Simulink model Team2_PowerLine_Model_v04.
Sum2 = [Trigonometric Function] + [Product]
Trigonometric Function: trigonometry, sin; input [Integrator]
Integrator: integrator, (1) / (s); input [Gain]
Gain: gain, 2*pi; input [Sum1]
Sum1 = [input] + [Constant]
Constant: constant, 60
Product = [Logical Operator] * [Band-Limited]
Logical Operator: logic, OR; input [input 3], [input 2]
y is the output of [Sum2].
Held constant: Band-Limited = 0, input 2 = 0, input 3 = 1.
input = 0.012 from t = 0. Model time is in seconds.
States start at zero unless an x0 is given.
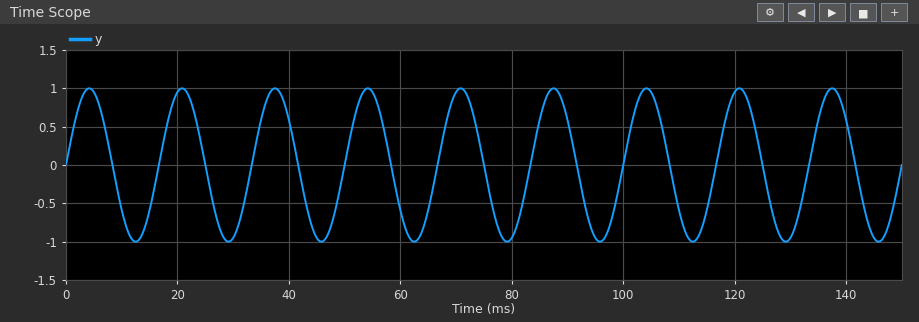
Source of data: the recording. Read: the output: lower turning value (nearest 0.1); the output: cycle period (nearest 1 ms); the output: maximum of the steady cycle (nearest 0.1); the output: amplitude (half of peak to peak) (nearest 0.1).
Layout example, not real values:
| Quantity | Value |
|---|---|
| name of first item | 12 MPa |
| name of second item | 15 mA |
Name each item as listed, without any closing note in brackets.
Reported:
| Quantity | Value |
|---|---|
| the output: lower turning value | -1.0 |
| the output: cycle period | 17 ms |
| the output: maximum of the steady cycle | 1.0 |
| the output: amplitude (half of peak to peak) | 1.0 |
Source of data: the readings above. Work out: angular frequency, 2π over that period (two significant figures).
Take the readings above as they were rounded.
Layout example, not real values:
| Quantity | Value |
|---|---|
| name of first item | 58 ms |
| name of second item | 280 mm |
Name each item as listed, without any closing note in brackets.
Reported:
| Quantity | Value |
|---|---|
| angular frequency, 2π over that period | 0.37 rad/ms |
